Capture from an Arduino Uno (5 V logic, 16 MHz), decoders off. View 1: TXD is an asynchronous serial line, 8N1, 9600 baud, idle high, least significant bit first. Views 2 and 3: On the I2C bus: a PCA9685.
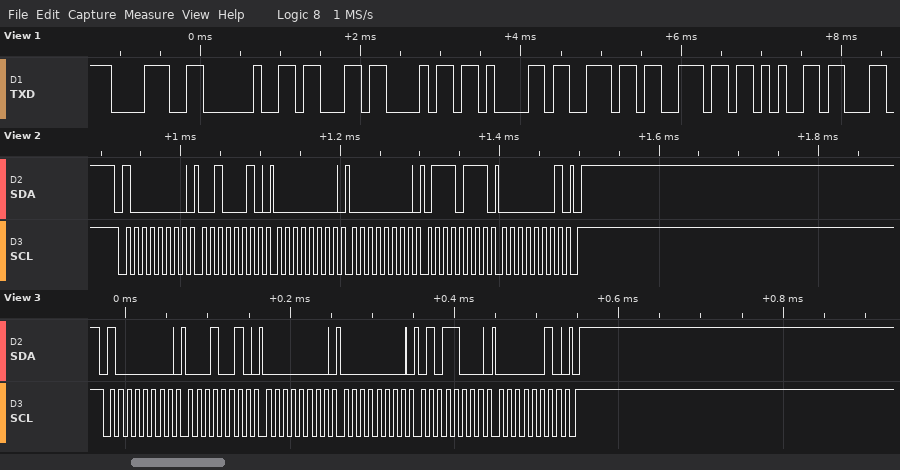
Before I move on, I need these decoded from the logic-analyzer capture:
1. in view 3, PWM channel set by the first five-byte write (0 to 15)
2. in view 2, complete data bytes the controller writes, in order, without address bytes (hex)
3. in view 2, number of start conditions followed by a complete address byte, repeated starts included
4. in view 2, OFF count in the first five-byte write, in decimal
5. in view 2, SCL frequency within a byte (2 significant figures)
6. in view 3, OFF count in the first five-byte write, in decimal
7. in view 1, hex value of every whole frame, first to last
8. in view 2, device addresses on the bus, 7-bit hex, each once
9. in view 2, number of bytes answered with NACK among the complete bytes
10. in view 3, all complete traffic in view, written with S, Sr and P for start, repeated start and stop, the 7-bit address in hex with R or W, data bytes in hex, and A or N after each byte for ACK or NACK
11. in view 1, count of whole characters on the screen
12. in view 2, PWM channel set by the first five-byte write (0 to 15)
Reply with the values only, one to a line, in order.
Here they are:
3
22 00 00 77 01
1
375
100 kHz
600
38 20 63 68 61 6E 6E 65
0x40
0
S 40W A 12 A 00 A 00 A 58 A 02 A P
8
7
